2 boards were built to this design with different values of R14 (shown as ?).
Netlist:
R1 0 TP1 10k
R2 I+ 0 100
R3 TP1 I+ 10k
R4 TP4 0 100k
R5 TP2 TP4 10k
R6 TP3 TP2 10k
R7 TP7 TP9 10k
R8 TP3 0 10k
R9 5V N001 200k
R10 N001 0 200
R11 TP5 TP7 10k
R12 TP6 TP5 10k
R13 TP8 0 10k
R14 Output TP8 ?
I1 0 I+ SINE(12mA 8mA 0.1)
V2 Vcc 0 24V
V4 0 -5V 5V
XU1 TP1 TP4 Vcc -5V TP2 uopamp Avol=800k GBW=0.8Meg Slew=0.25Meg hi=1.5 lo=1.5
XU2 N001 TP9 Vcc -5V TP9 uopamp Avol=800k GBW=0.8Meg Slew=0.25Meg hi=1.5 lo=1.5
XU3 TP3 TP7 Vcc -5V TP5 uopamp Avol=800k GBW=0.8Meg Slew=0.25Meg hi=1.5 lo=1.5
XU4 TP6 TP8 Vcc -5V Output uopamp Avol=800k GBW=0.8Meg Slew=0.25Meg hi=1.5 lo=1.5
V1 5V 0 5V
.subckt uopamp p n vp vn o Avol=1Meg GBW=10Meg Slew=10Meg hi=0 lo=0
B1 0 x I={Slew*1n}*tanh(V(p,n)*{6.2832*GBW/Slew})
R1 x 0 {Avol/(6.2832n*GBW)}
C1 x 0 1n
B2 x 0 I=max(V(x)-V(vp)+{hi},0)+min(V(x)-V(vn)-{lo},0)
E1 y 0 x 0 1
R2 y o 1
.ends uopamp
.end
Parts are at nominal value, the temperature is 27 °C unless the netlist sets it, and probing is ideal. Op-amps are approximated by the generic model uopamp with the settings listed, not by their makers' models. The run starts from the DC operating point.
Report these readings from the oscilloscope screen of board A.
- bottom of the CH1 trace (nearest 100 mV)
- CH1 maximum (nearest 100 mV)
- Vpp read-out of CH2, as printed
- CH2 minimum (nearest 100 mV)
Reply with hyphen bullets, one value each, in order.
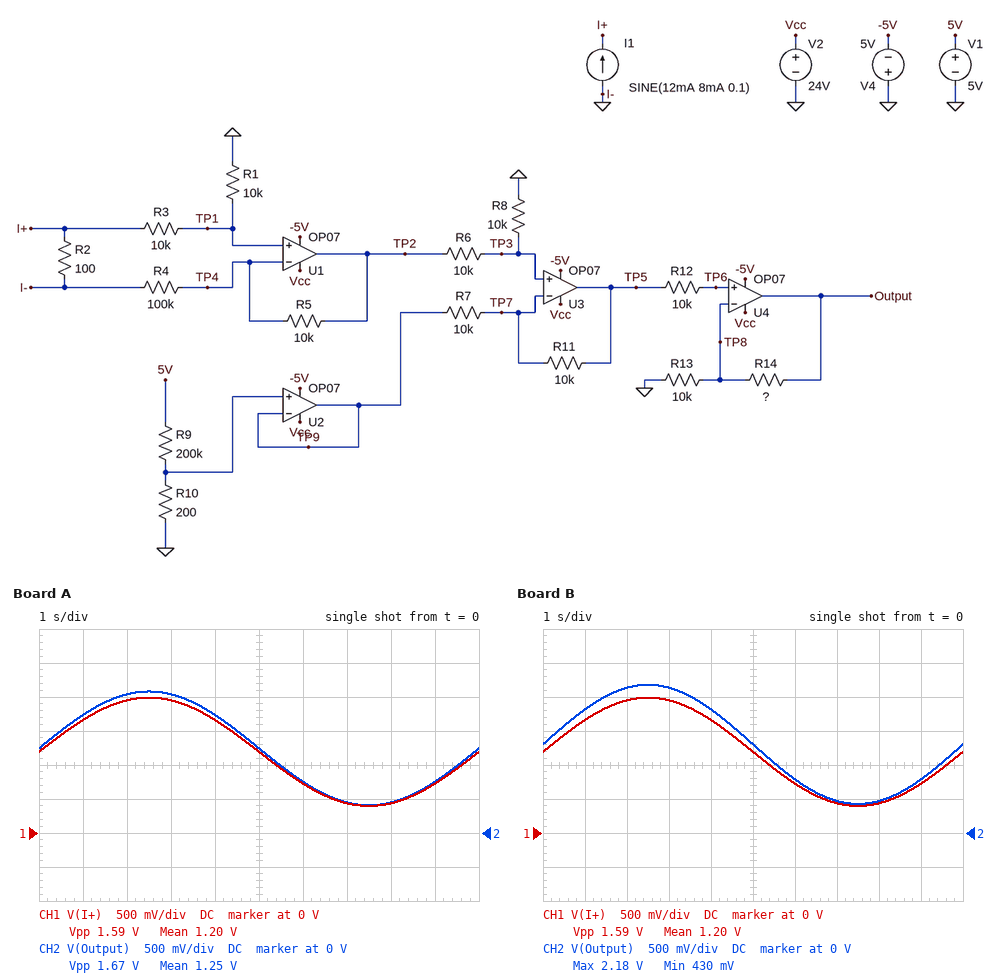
- 400 mV
- 2.0 V
- 1.67 V
- 400 mV
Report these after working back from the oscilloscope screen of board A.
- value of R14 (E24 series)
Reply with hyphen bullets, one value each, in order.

- 9.1 kΩ
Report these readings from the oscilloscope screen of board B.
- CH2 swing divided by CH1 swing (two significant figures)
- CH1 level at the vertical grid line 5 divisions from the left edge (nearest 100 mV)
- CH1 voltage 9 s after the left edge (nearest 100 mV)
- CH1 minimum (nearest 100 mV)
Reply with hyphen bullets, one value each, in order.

- 1.1
- 1.2 V
- 700 mV
- 400 mV
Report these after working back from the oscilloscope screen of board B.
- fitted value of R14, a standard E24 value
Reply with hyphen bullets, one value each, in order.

- 10 kΩ
